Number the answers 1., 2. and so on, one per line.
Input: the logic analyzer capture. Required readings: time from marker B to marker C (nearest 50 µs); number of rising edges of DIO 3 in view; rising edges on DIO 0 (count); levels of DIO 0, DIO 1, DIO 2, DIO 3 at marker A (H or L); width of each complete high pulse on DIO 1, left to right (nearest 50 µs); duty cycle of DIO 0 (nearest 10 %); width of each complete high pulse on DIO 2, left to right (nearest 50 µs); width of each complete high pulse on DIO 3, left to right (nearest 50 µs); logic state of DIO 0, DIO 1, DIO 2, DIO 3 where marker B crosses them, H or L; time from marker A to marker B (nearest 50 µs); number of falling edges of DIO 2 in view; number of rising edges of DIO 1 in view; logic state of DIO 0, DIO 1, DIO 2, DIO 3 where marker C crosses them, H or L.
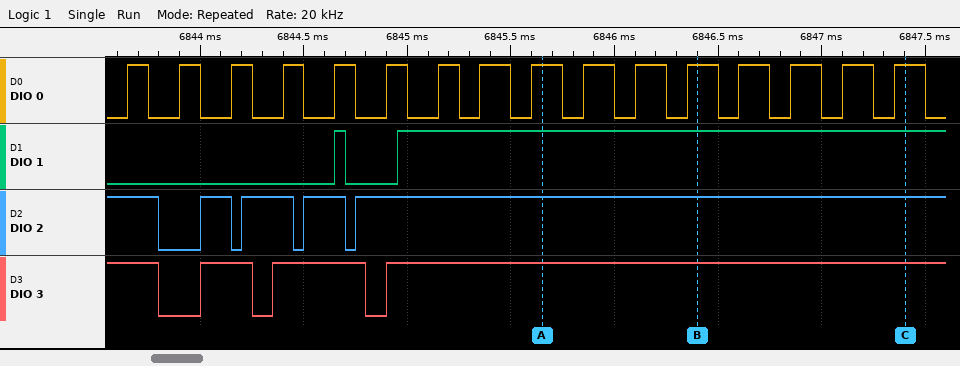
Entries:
1. 1000 µs
2. 3
3. 16
4. DIO 0=H, DIO 1=H, DIO 2=H, DIO 3=H
5. 50 µs
6. 50 %
7. 150 µs, 250 µs, 200 µs
8. 250 µs, 450 µs
9. DIO 0=H, DIO 1=H, DIO 2=H, DIO 3=H
10. 750 µs
11. 4
12. 2
13. DIO 0=H, DIO 1=H, DIO 2=H, DIO 3=H
